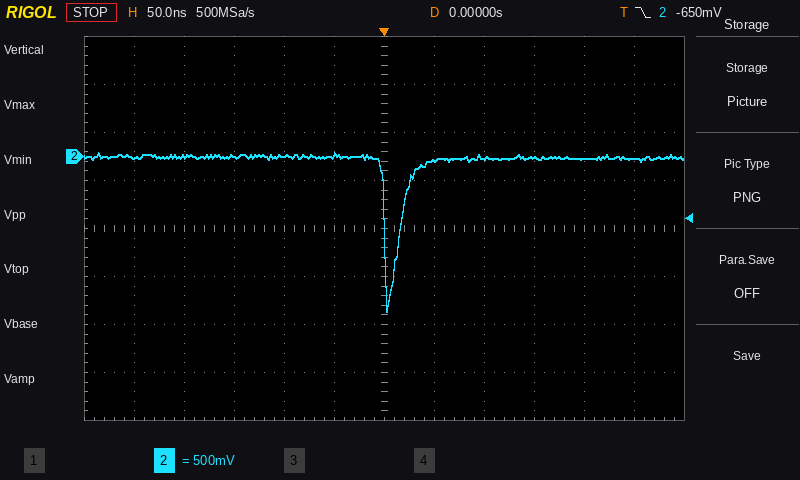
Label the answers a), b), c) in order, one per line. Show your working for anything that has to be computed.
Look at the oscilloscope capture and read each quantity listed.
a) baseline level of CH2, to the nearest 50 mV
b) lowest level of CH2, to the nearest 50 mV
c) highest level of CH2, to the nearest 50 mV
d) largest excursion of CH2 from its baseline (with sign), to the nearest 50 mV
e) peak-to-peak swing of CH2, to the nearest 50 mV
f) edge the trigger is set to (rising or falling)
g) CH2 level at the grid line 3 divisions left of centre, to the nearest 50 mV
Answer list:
a) 0 mV
b) -1.60 V
c) 50 mV
d) -1.60 V − (0 mV) = -1.60 V
e) 50 mV − (-1.60 V) = 1.65 V
f) falling
g) 0 mV
